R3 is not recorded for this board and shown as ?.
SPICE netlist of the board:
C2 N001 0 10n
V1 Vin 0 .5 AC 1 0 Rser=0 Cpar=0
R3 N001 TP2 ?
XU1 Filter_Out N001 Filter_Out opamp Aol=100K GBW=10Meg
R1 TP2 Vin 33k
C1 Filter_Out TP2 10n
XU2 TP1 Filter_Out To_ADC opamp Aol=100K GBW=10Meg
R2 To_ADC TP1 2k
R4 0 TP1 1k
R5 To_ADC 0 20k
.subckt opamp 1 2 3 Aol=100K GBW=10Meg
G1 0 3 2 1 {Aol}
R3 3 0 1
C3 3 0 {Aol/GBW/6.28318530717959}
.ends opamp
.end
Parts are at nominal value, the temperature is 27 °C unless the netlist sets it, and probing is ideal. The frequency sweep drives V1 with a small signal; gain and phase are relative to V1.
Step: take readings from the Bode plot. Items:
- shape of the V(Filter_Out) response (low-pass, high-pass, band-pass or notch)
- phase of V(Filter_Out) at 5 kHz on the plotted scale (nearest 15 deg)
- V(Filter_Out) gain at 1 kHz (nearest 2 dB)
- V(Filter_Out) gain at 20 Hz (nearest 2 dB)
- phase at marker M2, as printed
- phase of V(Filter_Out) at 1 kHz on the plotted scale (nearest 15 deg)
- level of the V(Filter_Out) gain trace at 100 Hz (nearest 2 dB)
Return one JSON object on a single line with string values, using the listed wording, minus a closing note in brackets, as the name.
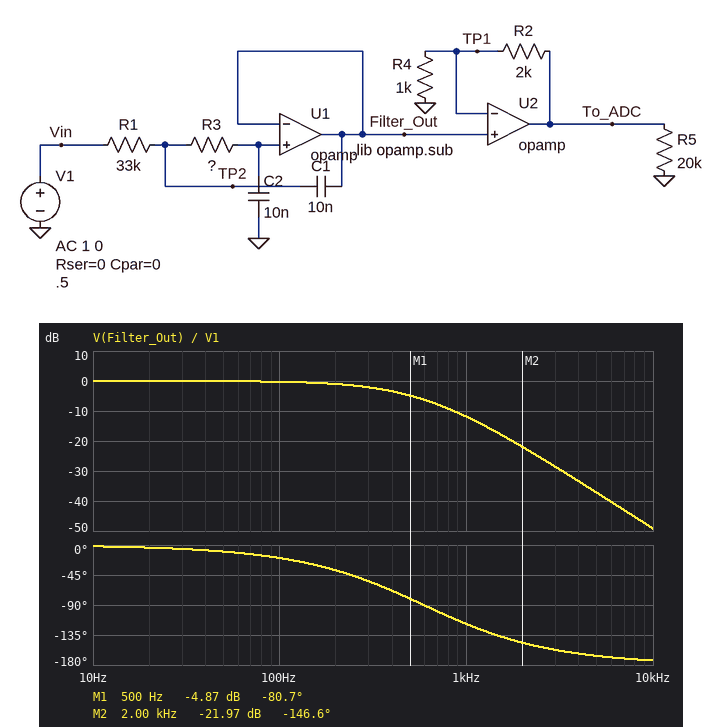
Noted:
{"shape of the V(Filter_Out) response": "low-pass", "phase of V(Filter_Out) at 5 kHz on the plotted scale": "-165 deg", "V(Filter_Out) gain at 1 kHz": "-12 dB", "V(Filter_Out) gain at 20 Hz": "0 dB", "phase at marker M2, as printed": "-146.6 deg", "phase of V(Filter_Out) at 1 kHz on the plotted scale": "-120 deg", "level of the V(Filter_Out) gain trace at 100 Hz": "0 dB"}
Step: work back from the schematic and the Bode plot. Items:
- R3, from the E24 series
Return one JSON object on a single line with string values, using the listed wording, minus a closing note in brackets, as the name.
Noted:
{"R3, from the E24 series": "22 kΩ"}
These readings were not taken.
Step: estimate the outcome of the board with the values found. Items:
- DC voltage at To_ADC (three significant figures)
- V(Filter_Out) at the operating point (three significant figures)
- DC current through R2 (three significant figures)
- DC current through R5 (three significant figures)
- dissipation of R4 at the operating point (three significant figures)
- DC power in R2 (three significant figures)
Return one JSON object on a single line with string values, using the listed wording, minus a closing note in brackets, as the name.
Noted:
{"DC voltage at To_ADC": "1.50 V", "V(Filter_Out) at the operating point": "500 mV", "DC current through R2": "500 µA", "DC current through R5": "75.0 µA", "dissipation of R4 at the operating point": "250 µW", "DC power in R2": "500 µW"}
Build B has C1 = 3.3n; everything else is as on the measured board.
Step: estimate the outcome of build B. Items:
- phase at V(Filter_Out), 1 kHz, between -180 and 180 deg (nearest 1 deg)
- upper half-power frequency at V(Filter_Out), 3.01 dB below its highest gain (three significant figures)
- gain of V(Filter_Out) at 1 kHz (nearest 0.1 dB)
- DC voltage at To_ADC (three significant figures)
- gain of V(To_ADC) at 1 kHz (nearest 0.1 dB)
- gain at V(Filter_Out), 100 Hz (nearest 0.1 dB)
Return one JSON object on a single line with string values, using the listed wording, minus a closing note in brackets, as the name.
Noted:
{"phase at V(Filter_Out), 1 kHz, between -180 and 180 deg": "-89 deg", "upper half-power frequency at V(Filter_Out), 3.01 dB below its highest gain": "314 Hz", "gain of V(Filter_Out) at 1 kHz": "-10.8 dB", "DC voltage at To_ADC": "1.50 V", "gain of V(To_ADC) at 1 kHz": "-1.2 dB", "gain at V(Filter_Out), 100 Hz": "-0.4 dB"}
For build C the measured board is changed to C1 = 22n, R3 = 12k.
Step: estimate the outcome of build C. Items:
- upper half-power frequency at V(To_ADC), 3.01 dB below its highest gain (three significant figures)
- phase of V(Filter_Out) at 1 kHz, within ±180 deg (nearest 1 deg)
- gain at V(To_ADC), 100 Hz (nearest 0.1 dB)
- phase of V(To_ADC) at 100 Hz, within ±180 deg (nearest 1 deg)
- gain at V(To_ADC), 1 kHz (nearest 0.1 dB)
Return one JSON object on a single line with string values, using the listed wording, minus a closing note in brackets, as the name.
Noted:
{"upper half-power frequency at V(To_ADC), 3.01 dB below its highest gain": "497 Hz", "phase of V(Filter_Out) at 1 kHz, within ±180 deg": "-131 deg", "gain at V(To_ADC), 100 Hz": "9.5 dB", "phase of V(To_ADC) at 100 Hz, within ±180 deg": "-16 deg", "gain at V(To_ADC), 1 kHz": "-1.9 dB"}
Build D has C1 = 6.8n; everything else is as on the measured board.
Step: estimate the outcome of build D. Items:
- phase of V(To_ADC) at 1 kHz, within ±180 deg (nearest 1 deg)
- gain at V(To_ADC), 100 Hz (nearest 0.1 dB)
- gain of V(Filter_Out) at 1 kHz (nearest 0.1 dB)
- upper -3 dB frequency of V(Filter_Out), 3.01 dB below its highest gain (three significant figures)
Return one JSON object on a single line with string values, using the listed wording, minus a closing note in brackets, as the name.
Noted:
{"phase of V(To_ADC) at 1 kHz, within ±180 deg": "-105 deg", "gain at V(To_ADC), 100 Hz": "9.2 dB", "gain of V(Filter_Out) at 1 kHz": "-11.1 dB", "upper -3 dB frequency of V(Filter_Out), 3.01 dB below its highest gain": "343 Hz"}
